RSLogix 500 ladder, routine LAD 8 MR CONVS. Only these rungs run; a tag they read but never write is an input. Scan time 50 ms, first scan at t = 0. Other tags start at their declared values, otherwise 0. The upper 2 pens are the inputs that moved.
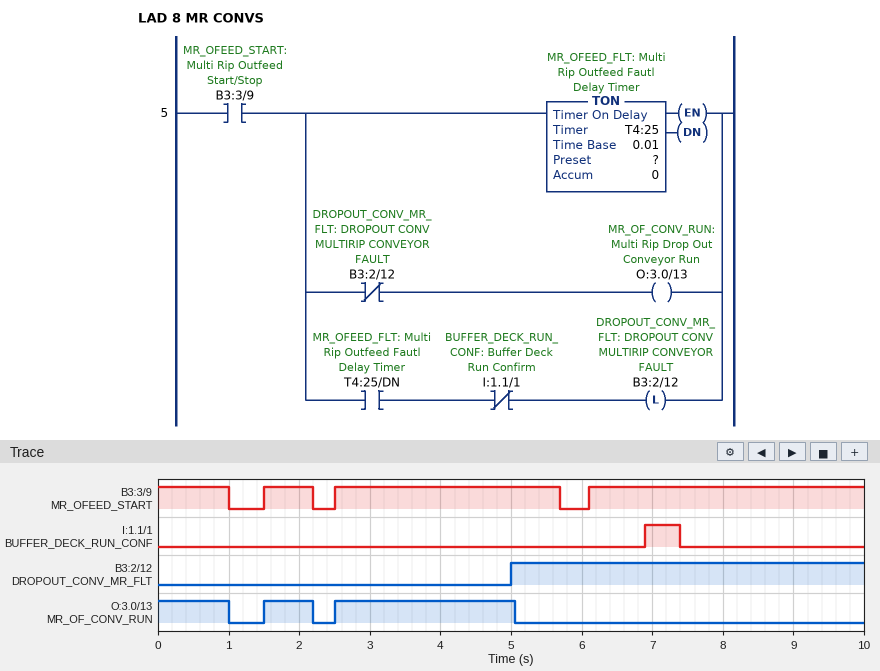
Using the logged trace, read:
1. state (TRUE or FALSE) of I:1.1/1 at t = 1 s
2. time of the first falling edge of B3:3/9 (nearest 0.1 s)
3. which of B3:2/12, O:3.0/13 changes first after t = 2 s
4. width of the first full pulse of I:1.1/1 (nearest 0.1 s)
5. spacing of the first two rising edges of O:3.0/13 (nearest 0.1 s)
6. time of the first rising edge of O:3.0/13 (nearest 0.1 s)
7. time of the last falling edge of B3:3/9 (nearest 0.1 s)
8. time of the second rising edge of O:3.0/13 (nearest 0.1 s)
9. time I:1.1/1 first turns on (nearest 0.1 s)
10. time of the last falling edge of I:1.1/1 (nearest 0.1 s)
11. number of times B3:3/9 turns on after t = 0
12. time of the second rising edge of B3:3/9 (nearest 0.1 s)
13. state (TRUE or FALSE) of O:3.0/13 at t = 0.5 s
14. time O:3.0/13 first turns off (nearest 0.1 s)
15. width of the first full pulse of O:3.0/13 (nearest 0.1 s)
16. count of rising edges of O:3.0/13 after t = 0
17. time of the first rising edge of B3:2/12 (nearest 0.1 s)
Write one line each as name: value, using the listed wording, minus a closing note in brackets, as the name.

state (TRUE or FALSE) of I:1.1/1 at t = 1 s: FALSE
time of the first falling edge of B3:3/9: 1.0 s
which of B3:2/12, O:3.0/13 changes first after t = 2 s: O:3.0/13
width of the first full pulse of I:1.1/1: 0.5 s
spacing of the first two rising edges of O:3.0/13: 1.0 s
time of the first rising edge of O:3.0/13: 1.5 s
time of the last falling edge of B3:3/9: 5.7 s
time of the second rising edge of O:3.0/13: 2.5 s
time I:1.1/1 first turns on: 6.9 s
time of the last falling edge of I:1.1/1: 7.4 s
number of times B3:3/9 turns on after t = 0: 3
time of the second rising edge of B3:3/9: 2.5 s
state (TRUE or FALSE) of O:3.0/13 at t = 0.5 s: TRUE
time O:3.0/13 first turns off: 1.0 s
width of the first full pulse of O:3.0/13: 0.7 s
count of rising edges of O:3.0/13 after t = 0: 2
time of the first rising edge of B3:2/12: 5.0 s
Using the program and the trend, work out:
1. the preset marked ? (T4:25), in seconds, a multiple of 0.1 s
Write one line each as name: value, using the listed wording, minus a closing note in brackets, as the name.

the preset marked ? (T4:25), in seconds, a multiple of 0.1 s: 2.5 s
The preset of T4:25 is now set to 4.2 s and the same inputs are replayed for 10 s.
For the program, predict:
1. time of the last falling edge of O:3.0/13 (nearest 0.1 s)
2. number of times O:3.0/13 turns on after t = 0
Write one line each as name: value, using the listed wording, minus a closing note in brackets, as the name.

time of the last falling edge of O:3.0/13: 5.7 s
number of times O:3.0/13 turns on after t = 0: 3
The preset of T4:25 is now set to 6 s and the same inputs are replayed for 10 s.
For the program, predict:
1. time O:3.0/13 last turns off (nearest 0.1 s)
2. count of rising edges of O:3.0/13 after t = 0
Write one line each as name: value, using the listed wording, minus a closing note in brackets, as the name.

time O:3.0/13 last turns off: 5.7 s
count of rising edges of O:3.0/13 after t = 0: 3
